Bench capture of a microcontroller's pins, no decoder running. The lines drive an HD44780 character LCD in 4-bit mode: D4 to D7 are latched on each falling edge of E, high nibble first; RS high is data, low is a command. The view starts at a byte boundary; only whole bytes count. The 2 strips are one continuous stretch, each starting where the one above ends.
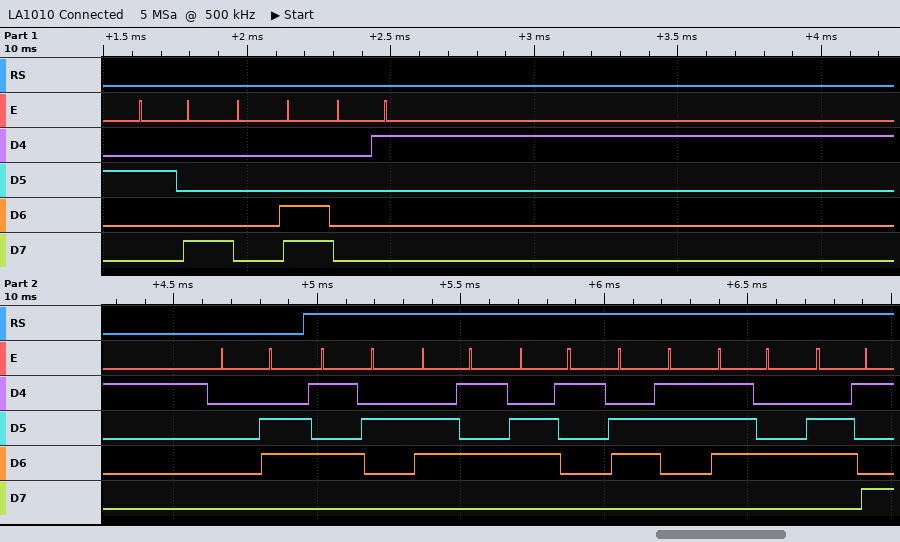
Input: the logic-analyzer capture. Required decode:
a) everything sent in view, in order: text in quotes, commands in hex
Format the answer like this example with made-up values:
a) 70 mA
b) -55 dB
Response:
a) 0x28 0x0C 0x01 0x06 "Reacti"
